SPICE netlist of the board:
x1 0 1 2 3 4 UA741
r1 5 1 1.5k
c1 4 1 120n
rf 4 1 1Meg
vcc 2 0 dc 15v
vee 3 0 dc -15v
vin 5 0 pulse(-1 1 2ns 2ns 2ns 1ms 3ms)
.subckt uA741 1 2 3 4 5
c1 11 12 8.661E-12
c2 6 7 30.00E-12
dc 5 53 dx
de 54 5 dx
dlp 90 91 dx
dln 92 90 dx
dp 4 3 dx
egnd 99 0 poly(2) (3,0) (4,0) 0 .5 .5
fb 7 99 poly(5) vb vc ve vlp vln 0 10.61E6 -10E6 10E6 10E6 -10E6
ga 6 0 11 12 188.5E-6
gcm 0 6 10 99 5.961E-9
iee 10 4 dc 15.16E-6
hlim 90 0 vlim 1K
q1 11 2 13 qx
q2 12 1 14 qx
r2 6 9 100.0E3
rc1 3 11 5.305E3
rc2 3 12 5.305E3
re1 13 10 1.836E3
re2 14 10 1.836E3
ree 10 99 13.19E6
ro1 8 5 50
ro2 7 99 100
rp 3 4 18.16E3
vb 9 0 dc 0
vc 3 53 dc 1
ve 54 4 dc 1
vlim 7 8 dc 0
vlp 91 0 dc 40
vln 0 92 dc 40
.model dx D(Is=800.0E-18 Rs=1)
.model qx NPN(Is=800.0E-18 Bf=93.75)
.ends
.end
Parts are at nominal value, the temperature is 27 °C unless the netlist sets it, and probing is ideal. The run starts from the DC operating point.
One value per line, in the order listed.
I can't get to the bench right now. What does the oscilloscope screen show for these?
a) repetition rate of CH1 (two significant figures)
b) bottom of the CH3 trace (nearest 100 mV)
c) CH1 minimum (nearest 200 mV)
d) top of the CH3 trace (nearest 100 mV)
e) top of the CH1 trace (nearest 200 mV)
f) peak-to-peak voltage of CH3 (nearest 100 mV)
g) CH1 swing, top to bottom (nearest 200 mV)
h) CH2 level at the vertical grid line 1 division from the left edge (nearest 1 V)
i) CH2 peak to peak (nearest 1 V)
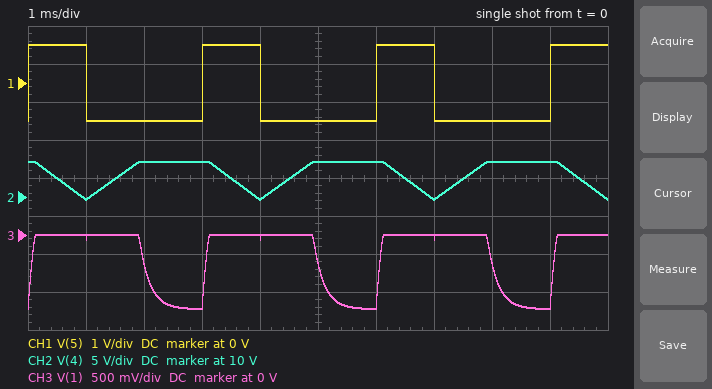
330 Hz
-1.0 V
-1.0 V
0 V
1.0 V
1.0 V
2.0 V
10 V
5 V
